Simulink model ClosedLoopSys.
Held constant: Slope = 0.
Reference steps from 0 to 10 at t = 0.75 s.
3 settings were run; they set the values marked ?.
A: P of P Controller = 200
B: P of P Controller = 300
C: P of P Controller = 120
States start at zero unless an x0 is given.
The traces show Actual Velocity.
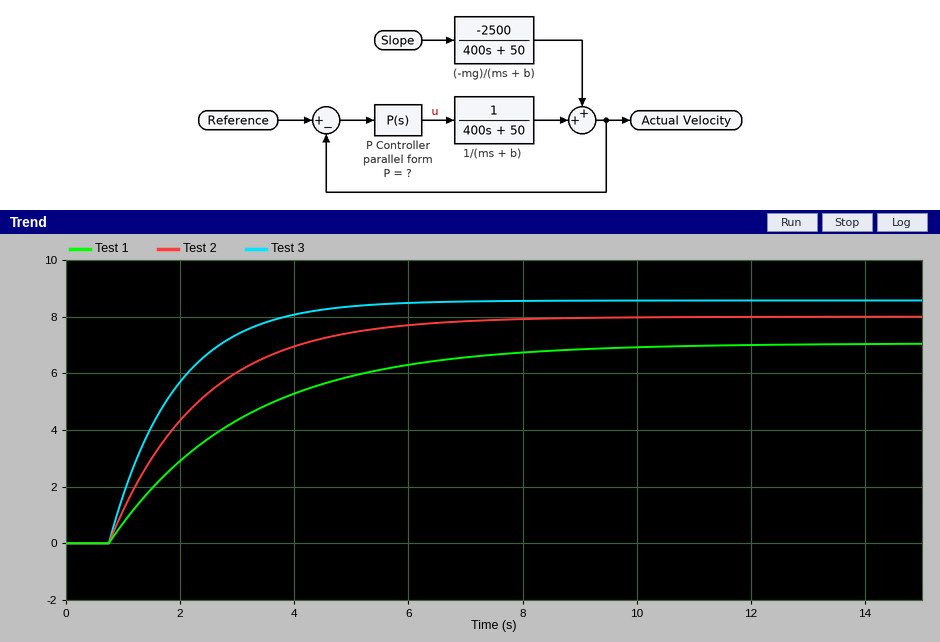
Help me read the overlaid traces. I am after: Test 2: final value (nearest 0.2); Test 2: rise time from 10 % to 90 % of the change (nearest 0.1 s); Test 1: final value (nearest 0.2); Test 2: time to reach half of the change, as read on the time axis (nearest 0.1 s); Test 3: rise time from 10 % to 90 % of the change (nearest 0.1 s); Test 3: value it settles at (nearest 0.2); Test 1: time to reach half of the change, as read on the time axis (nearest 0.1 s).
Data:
8.0
3.5 s
7.0
1.9 s
2.5 s
8.6
2.4 s
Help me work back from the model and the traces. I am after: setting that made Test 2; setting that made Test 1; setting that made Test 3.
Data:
A
C
B
